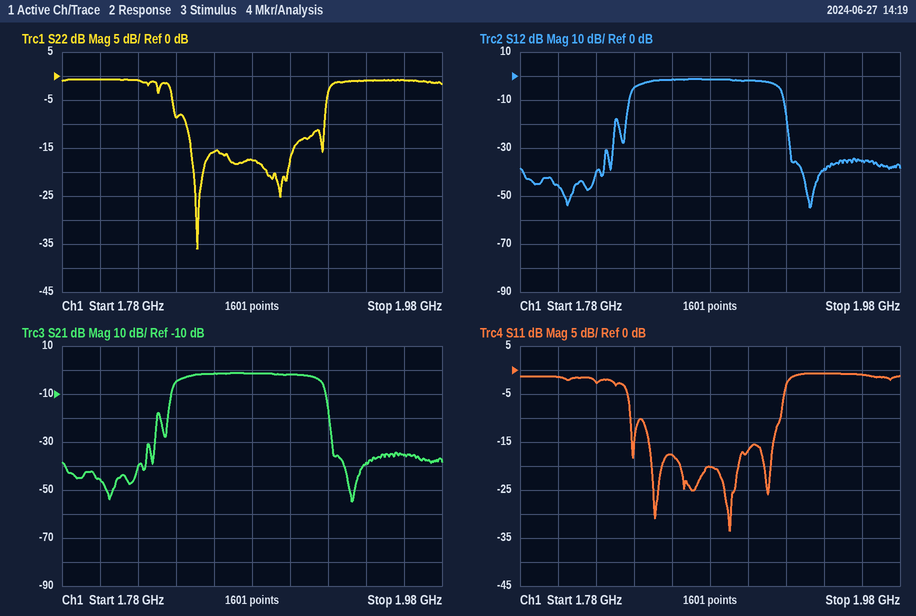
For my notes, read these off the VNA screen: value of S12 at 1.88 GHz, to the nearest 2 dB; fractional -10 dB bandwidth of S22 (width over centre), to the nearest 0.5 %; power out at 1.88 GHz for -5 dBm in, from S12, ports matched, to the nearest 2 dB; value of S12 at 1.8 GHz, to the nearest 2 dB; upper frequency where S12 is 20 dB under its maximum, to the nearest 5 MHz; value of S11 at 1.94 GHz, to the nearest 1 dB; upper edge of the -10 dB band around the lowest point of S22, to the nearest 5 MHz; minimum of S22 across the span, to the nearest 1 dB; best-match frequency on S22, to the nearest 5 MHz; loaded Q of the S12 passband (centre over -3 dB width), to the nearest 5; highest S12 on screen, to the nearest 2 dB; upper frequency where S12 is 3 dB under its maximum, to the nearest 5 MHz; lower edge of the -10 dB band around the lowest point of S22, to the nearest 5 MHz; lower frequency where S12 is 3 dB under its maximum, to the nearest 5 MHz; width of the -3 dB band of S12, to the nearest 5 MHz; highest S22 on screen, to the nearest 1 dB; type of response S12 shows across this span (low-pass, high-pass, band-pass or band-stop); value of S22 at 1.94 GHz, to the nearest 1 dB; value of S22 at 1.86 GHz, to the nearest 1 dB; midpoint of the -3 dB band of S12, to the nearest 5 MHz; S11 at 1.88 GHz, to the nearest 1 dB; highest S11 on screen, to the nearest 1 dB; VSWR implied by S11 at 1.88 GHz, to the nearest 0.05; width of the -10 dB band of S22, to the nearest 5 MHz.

-2 dB
4.0 %
-6 dBm
-46 dB
1.920 GHz
-1 dB
1.920 GHz
-36 dB
1.850 GHz
25
-2 dB
1.915 GHz
1.845 GHz
1.840 GHz
75 MHz
-1 dB
band-pass
-1 dB
-16 dB
1.880 GHz
-20 dB
-1 dB
1.20
75 MHz
